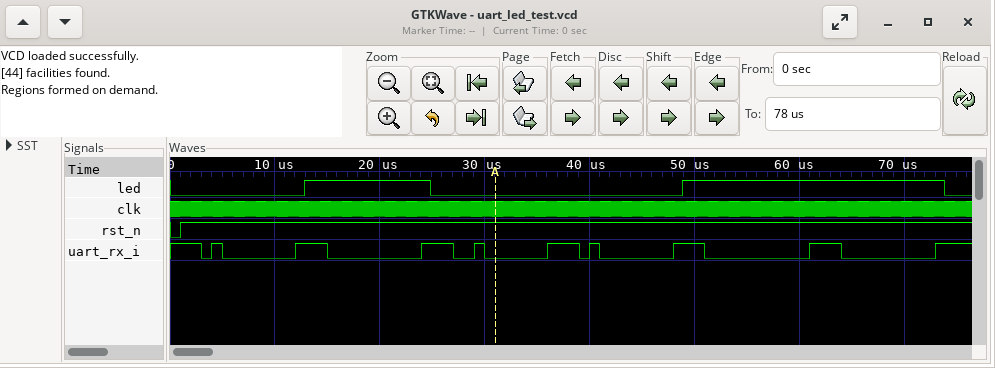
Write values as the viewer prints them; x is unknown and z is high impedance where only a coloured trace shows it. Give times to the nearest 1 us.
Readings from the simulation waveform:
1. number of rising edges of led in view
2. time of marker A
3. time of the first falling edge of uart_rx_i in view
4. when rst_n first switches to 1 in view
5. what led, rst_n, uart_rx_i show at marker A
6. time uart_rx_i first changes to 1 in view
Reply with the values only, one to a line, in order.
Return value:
2
31 us
3 us
1 us
led=0, rst_n=1, uart_rx_i=0
4 us
